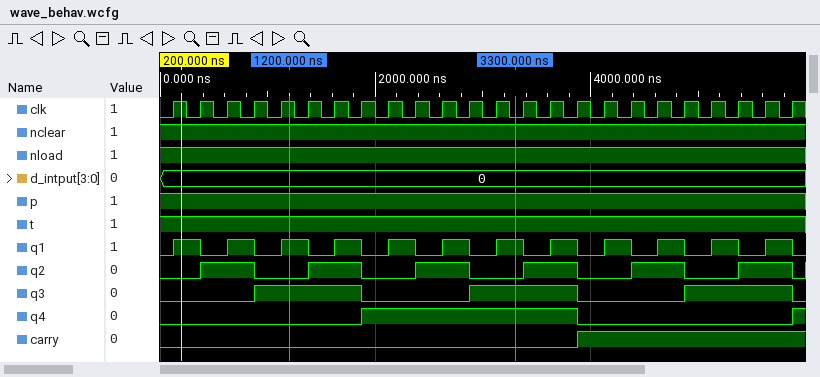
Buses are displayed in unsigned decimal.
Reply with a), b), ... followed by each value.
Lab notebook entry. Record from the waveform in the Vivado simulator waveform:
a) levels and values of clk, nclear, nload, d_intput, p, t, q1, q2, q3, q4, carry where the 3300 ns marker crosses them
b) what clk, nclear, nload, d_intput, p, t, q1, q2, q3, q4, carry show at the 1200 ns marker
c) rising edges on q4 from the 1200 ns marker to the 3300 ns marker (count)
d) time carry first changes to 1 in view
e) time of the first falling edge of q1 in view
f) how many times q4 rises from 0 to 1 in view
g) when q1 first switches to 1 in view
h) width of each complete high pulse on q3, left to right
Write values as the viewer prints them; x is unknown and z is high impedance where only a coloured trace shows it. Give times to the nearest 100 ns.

a) clk=0, nclear=1, nload=1, d_intput=0, p=1, t=1, q1=1, q2=0, q3=1, q4=1, carry=0
b) clk=1, nclear=1, nload=1, d_intput=0, p=1, t=1, q1=1, q2=0, q3=1, q4=0, carry=0
c) 1
d) 3900 ns
e) 400 ns
f) 2
g) 100 ns
h) 1000 ns, 1000 ns, 1000 ns
